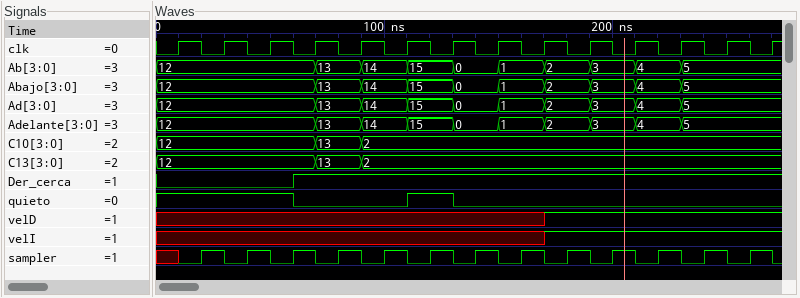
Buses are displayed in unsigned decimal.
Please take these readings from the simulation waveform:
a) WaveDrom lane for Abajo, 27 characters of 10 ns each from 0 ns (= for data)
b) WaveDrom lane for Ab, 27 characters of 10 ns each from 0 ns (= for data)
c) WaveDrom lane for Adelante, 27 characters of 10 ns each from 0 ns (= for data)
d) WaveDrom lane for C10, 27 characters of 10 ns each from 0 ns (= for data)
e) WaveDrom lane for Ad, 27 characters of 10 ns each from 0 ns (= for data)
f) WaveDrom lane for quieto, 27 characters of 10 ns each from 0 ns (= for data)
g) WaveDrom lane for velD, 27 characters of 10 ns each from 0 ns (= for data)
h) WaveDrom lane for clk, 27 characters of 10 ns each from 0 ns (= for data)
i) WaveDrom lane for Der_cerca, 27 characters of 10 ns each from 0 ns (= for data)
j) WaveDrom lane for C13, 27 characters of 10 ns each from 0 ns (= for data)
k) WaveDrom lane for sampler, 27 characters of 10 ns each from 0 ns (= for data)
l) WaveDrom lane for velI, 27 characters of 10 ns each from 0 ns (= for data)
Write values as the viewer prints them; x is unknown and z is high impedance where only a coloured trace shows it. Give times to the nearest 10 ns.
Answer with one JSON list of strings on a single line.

["{name: 'Abajo', wave: '=......=.=.=.=.=.=.=.=.=...', data: '12 13 14 15 0 1 2 3 4 5'}", "{name: 'Ab', wave: '=......=.=.=.=.=.=.=.=.=...', data: '12 13 14 15 0 1 2 3 4 5'}", "{name: 'Adelante', wave: '=......=.=.=.=.=.=.=.=.=...', data: '12 13 14 15 0 1 2 3 4 5'}", "{name: 'C10', wave: '=......=.=.................', data: '12 13 2'}", "{name: 'Ad', wave: '=......=.=.=.=.=.=.=.=.=...', data: '12 13 14 15 0 1 2 3 4 5'}", "{name: 'quieto', wave: '1.....0....1.0.............'}", "{name: 'velD', wave: 'x................1.........'}", "{name: 'clk', wave: '010101010101010101010101010'}", "{name: 'Der_cerca', wave: '0.....1....................'}", "{name: 'C13', wave: '=......=.=.................', data: '12 13 2'}", "{name: 'sampler', wave: 'x01010101010101010101010101'}", "{name: 'velI', wave: 'x................1.........'}"]
